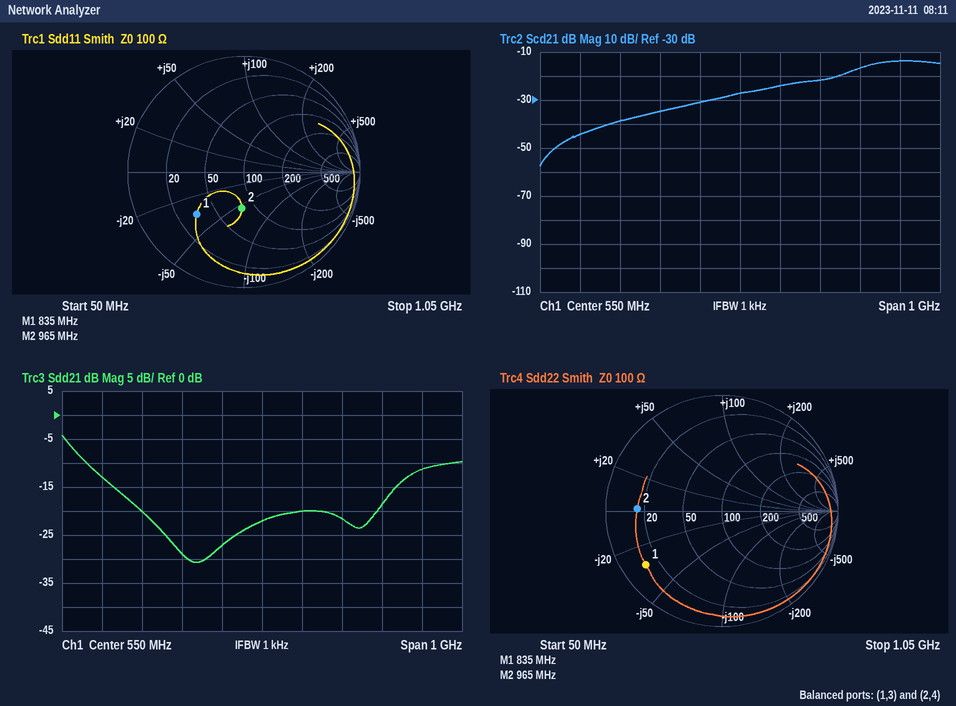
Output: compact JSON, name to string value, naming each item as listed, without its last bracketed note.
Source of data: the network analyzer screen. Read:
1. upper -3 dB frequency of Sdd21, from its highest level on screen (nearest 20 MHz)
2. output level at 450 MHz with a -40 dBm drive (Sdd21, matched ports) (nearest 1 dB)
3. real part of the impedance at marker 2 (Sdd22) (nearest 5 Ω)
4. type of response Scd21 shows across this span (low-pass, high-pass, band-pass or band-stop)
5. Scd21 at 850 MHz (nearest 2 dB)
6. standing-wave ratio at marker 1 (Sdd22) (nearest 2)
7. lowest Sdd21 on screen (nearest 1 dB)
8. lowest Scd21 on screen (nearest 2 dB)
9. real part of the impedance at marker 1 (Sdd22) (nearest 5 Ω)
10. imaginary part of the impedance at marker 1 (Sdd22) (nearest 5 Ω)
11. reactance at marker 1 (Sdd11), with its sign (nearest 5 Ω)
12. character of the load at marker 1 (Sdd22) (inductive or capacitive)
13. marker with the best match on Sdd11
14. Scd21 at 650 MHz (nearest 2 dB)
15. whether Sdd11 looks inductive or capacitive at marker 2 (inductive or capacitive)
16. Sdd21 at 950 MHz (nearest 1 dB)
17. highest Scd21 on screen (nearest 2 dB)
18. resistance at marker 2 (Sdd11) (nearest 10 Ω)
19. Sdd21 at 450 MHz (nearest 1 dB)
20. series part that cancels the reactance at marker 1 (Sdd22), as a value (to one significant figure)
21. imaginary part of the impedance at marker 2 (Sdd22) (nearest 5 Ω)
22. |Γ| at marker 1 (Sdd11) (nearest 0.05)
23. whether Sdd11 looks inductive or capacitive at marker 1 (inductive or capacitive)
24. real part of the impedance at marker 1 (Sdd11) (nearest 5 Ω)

{"upper -3 dB frequency of Sdd21, from its highest level on screen": "80 MHz", "output level at 450 MHz with a -40 dBm drive (Sdd21, matched ports)": "-67 dBm", "real part of the impedance at marker 2 (Sdd22)": "15 Ω", "type of response Scd21 shows across this span": "high-pass", "Scd21 at 850 MHz": "-16 dB", "standing-wave ratio at marker 1 (Sdd22)": "10", "lowest Sdd21 on screen": "-31 dB", "lowest Scd21 on screen": "-58 dB", "real part of the impedance at marker 1 (Sdd22)": "10 Ω", "imaginary part of the impedance at marker 1 (Sdd22)": "-30 Ω", "reactance at marker 1 (Sdd11), with its sign": "-35 Ω", "character of the load at marker 1 (Sdd22)": "capacitive", "marker with the best match on Sdd11": "marker 2", "Scd21 at 650 MHz": "-24 dB", "whether Sdd11 looks inductive or capacitive at marker 2": "capacitive", "Sdd21 at 950 MHz": "-11 dB", "highest Scd21 on screen": "-14 dB", "resistance at marker 2 (Sdd11)": "80 Ω", "Sdd21 at 450 MHz": "-27 dB", "series part that cancels the reactance at marker 1 (Sdd22), as a value": "6 nH", "imaginary part of the impedance at marker 2 (Sdd22)": "0 Ω", "|Γ| at marker 1 (Sdd11)": "0.55", "whether Sdd11 looks inductive or capacitive at marker 1": "capacitive", "real part of the impedance at marker 1 (Sdd11)": "35 Ω"}
